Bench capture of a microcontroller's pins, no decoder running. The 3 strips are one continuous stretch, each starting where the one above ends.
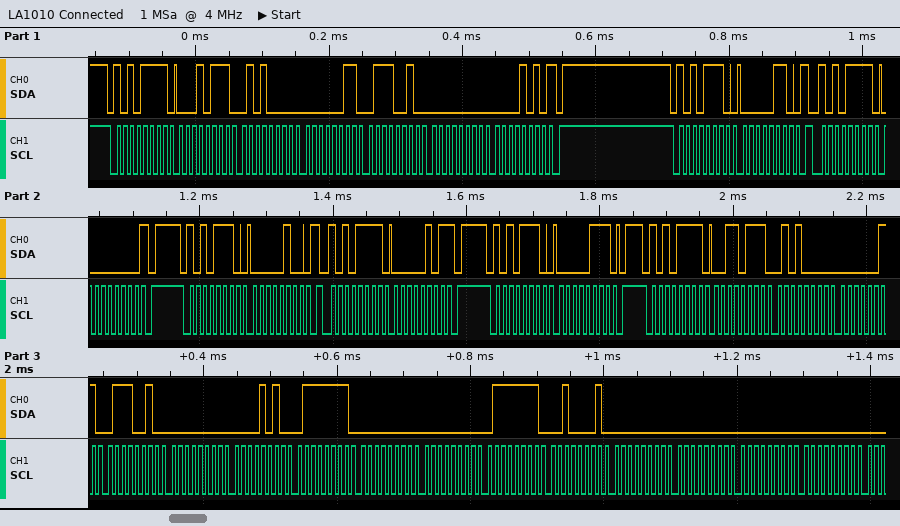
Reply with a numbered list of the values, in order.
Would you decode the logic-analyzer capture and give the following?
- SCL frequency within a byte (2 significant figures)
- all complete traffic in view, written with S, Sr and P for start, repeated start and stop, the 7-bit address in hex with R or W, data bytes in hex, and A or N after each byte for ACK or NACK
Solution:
1. 100 kHz
2. S 57R A 17 A 50 A 03 A 72 A 00 A 0A N P S 57W A 06 A Sr 57R A 00 N P S 57W A 04 A Sr 57R A 05 N P S 57W A 07 A P S 57R A 37 A 50 A 03 A 72 A 00 A 0A A 7F A 00 A 00 A 7F A 21 A 00 A 00 A 00 A 00 A
